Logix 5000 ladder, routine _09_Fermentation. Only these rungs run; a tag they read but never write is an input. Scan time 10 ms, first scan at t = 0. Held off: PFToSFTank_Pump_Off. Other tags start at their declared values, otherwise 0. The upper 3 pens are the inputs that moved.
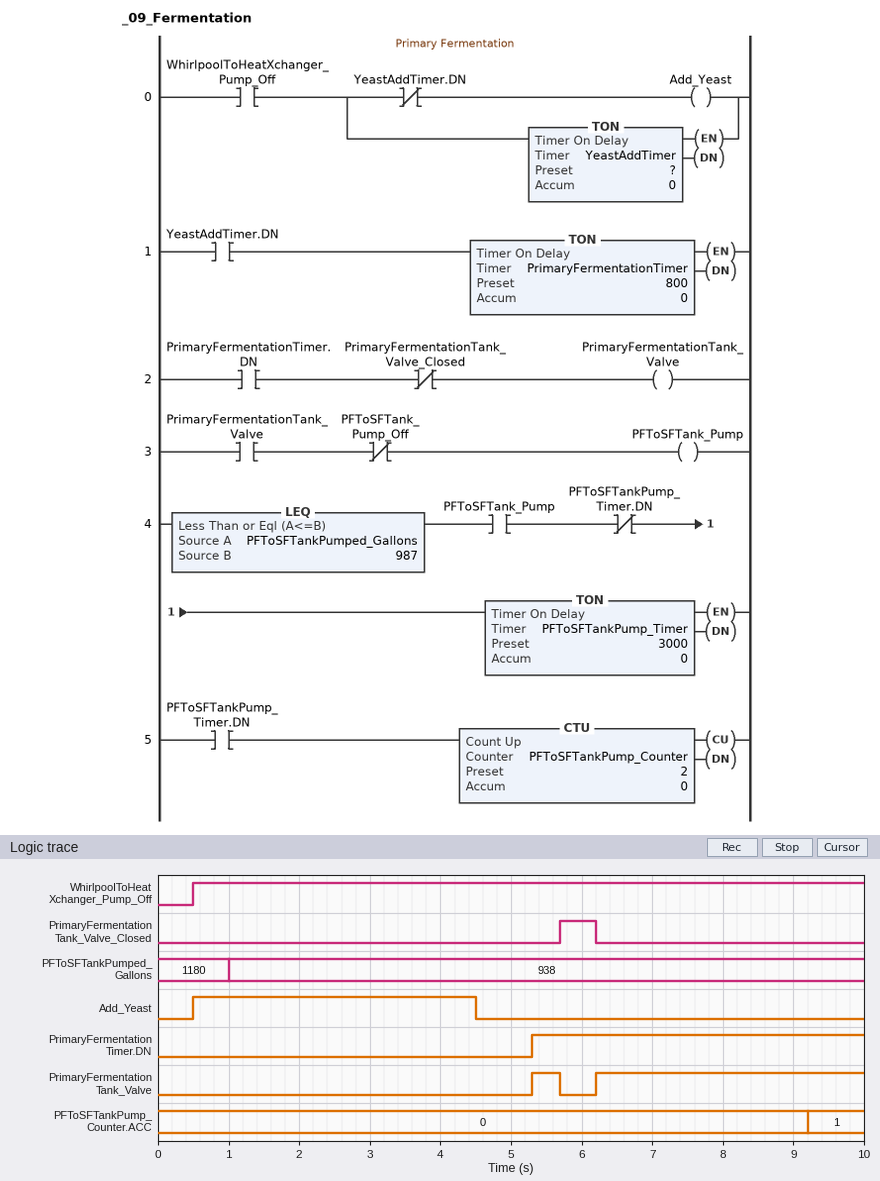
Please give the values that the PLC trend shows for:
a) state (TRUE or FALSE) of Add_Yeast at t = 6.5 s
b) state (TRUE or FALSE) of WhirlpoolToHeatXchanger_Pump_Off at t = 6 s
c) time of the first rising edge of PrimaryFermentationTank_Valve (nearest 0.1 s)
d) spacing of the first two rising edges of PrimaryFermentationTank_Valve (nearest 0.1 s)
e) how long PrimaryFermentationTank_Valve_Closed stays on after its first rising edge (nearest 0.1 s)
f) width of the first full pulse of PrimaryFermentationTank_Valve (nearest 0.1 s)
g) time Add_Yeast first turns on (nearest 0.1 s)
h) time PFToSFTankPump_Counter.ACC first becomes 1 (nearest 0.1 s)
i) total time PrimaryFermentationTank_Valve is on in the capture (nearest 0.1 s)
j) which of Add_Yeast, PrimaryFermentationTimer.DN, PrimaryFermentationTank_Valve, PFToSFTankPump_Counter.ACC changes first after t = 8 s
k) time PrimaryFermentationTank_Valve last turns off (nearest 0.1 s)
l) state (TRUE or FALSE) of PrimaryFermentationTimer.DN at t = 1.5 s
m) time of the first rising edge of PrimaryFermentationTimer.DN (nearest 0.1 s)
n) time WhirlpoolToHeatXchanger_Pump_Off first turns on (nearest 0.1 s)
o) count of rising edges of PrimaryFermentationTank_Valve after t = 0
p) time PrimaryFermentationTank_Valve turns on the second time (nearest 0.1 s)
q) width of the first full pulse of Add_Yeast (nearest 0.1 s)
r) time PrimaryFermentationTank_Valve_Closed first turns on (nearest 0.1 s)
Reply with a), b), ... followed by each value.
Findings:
a) FALSE
b) TRUE
c) 5.3 s
d) 0.9 s
e) 0.5 s
f) 0.4 s
g) 0.5 s
h) 9.2 s
i) 4.2 s
j) PFToSFTankPump_Counter.ACC
k) 5.7 s
l) FALSE
m) 5.3 s
n) 0.5 s
o) 2
p) 6.2 s
q) 4.0 s
r) 5.7 s
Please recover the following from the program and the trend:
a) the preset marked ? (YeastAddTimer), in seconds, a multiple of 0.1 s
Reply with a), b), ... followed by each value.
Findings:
a) 4.0 s
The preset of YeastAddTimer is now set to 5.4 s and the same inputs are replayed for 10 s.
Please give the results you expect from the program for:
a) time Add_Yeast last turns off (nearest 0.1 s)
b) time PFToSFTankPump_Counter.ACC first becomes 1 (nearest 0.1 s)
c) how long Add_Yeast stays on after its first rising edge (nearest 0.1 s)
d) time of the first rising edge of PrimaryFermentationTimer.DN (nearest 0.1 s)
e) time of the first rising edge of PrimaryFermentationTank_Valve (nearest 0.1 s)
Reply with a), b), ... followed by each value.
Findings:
a) 5.9 s
b) 9.7 s
c) 5.4 s
d) 6.7 s
e) 6.7 s
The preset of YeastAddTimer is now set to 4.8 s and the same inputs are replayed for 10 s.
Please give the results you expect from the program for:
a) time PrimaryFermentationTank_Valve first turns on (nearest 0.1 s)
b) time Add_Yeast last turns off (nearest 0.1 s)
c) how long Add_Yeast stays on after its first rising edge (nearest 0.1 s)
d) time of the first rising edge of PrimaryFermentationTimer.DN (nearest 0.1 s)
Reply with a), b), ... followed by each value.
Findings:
a) 6.2 s
b) 5.3 s
c) 4.8 s
d) 6.1 s
